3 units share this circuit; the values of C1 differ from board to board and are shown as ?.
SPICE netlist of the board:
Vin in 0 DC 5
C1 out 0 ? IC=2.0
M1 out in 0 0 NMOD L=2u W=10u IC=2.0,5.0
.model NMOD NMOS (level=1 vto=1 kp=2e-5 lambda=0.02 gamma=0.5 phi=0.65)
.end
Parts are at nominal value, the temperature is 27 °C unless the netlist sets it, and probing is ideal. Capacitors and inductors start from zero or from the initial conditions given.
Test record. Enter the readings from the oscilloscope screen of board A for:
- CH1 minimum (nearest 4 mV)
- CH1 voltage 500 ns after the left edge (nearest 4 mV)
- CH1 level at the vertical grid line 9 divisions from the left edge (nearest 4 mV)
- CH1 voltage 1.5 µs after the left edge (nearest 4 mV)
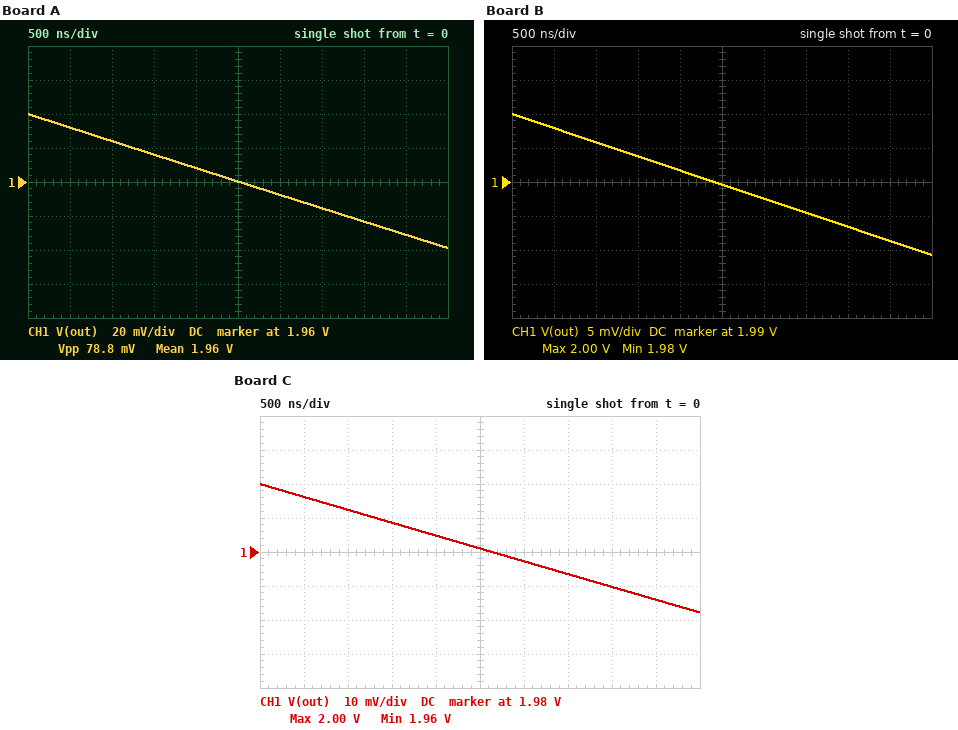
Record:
1.920 V
1.992 V
1.928 V
1.976 V
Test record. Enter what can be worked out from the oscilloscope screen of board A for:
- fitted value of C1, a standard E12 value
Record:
39 nF
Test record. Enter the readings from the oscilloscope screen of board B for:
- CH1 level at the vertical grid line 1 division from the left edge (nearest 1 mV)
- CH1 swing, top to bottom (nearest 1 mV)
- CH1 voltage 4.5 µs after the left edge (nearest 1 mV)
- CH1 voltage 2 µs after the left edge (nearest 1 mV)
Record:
1.998 V
21 mV
1.981 V
1.992 V
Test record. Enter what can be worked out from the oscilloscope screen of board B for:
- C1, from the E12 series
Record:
150 nF
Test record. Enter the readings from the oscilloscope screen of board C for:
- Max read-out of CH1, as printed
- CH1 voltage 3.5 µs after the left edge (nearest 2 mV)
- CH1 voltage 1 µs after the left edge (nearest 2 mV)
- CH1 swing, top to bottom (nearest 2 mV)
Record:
2.00 V
1.974 V
1.992 V
38 mV
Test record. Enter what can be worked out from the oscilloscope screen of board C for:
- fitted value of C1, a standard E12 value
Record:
82 nF
